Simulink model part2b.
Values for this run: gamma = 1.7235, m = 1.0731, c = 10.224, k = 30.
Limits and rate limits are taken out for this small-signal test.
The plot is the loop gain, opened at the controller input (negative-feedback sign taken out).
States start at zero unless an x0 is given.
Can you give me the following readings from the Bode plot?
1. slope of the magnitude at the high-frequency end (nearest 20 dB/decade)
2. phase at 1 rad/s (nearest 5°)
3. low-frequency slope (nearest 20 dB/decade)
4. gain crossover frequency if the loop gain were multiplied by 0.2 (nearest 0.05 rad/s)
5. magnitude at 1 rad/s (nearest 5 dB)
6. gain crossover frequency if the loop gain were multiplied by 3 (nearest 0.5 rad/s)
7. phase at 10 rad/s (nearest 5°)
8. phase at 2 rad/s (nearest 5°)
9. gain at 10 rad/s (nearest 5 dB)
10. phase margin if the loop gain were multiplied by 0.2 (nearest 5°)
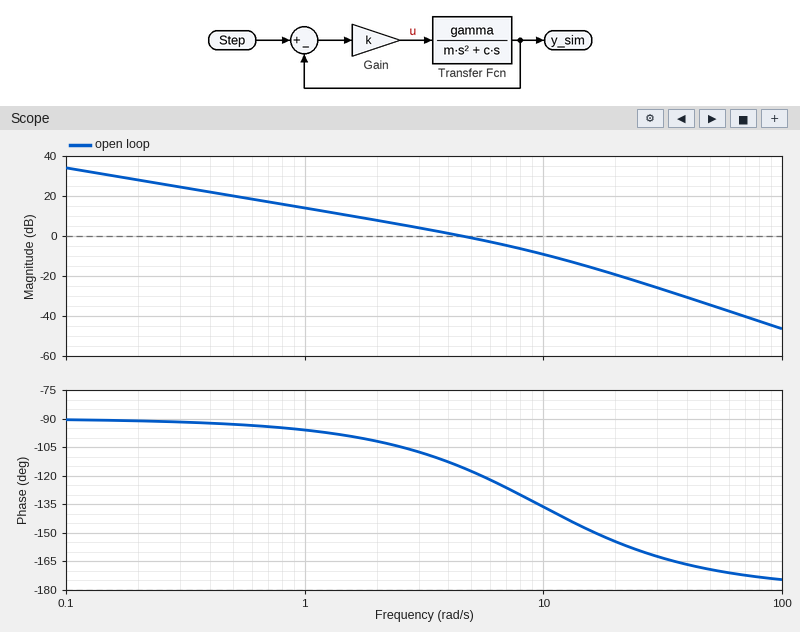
-40 dB/decade
-95°
-20 dB/decade
1.00 rad/s
15 dB
10.5 rad/s
-135°
-100°
-10 dB
85°
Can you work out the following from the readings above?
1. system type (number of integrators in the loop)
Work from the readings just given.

1
